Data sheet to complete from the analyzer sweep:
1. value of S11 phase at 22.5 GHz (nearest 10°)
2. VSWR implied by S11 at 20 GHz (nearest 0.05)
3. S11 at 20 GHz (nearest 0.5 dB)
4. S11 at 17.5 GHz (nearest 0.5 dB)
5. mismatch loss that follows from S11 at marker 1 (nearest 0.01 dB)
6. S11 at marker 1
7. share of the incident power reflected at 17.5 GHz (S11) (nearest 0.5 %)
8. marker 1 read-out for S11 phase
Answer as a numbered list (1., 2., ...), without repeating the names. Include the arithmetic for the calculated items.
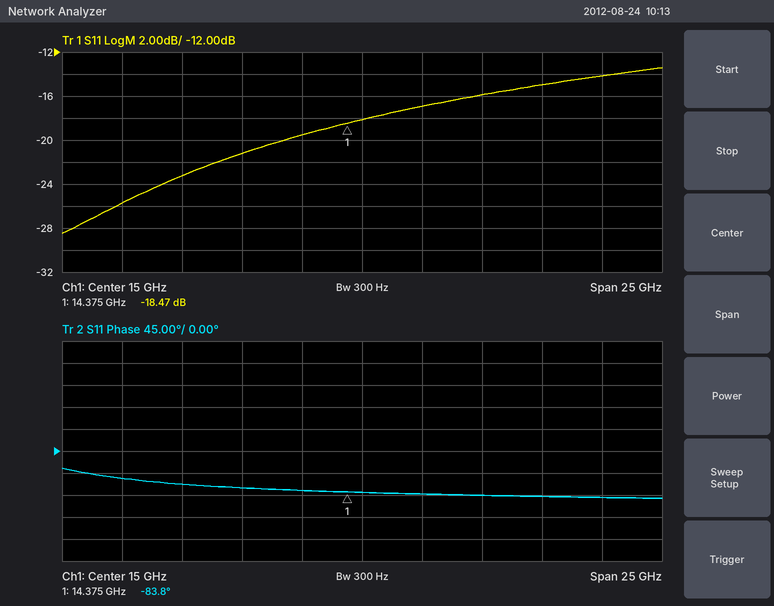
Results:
1. -90°
2. |Γ| = 10^(-16/20) = 0.1585; VSWR = (1 + 0.1585)/(1 − 0.1585) ≈ 1.38, so 1.40 to the nearest 0.05
3. -16.0 dB
4. -17.0 dB
5. −10 log10(1 − 10^(-18.47/10)) ≈ 0.06 dB
6. -18.47 dB
7. 10^(-17/10) ≈ 2.0 %
8. -83.8°
